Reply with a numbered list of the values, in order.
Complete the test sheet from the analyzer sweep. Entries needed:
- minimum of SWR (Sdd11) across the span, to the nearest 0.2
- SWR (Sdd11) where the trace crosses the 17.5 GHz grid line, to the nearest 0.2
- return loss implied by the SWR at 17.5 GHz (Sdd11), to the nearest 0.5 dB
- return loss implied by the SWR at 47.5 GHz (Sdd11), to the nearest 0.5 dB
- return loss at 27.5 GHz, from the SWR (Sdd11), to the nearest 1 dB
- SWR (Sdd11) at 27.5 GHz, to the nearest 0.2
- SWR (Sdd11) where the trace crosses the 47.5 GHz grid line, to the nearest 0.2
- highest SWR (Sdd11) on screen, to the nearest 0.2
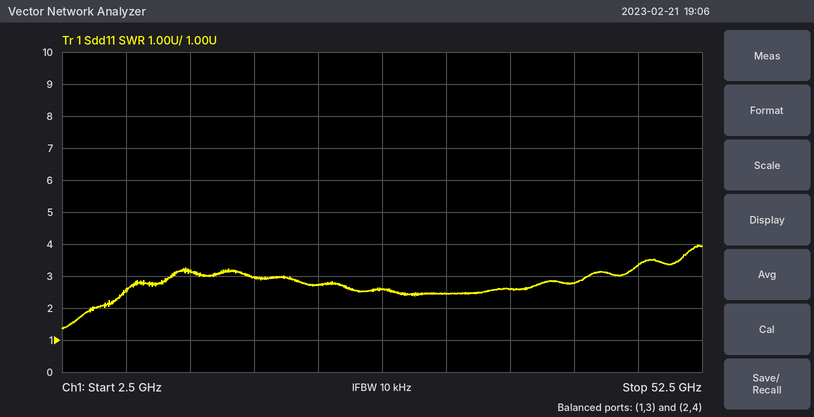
1. 1.4
2. 3.0
3. 6.0 dB
4. 5.5 dB
5. 7 dB
6. 2.6
7. 3.4
8. 4.0
